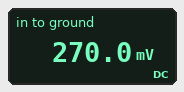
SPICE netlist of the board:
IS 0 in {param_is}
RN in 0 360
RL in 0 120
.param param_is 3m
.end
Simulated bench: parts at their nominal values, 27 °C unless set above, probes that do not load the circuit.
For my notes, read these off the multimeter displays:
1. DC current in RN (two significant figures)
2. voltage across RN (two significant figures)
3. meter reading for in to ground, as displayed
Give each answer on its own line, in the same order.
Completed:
750 µA
270 mV
270.0 mV
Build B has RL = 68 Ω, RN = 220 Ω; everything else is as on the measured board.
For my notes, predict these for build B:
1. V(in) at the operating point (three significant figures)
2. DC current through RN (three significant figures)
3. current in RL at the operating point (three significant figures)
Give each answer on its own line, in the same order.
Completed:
156 mV
708 µA
2.29 mA
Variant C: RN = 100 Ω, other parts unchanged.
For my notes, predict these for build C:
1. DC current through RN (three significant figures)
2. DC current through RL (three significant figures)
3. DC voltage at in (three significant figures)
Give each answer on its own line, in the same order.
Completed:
1.64 mA
1.36 mA
164 mV
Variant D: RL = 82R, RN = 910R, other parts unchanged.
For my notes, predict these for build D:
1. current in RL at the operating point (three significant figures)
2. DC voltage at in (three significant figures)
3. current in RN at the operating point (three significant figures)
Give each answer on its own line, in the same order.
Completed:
2.75 mA
226 mV
248 µA
